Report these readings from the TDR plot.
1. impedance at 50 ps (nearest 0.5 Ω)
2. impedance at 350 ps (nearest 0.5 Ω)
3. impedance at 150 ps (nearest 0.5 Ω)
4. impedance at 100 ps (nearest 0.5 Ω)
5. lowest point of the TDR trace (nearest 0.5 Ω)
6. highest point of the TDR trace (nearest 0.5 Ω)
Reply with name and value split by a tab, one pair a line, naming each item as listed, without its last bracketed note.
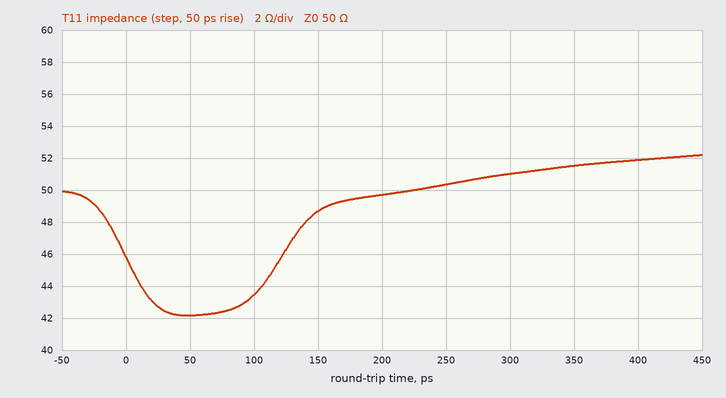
impedance at 50 ps	42.0 Ω
impedance at 350 ps	51.5 Ω
impedance at 150 ps	48.5 Ω
impedance at 100 ps	43.5 Ω
lowest point of the TDR trace	42.0 Ω
highest point of the TDR trace	52.0 Ω
